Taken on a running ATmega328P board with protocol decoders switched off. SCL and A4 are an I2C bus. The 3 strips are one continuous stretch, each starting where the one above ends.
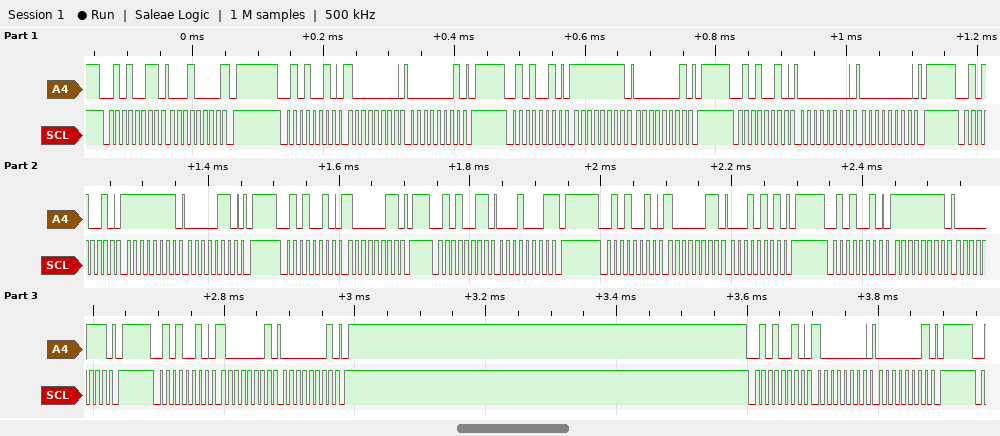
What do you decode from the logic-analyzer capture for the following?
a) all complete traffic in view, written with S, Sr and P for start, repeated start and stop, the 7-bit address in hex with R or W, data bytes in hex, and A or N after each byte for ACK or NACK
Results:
S 29R A 10 N P S 29W A 80 A 01 A P S 29W A FF A 01 A P S 29W A 00 A 00 A P S 29W A FF A 06 A P S 29W A 83 A P S 29R A 11 N P S 29W A 83 A 15 A P S 29W A FF A 07 A P S 29W A 81 A 01 A P S 29W A 80 A 01 A P
